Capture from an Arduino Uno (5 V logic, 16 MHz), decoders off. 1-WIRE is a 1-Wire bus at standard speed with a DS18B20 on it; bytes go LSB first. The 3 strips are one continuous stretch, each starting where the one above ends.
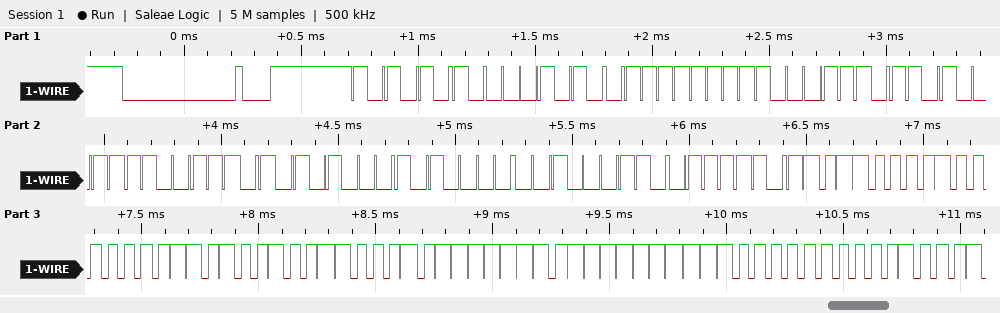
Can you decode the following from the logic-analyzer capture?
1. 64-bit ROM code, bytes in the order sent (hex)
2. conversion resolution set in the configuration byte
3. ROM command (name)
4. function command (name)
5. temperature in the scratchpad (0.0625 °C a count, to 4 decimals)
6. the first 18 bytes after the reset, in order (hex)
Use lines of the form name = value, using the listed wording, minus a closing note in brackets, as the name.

64-bit ROM code, bytes in the order sent = 28 FF 71 CB 73 15 05 62
conversion resolution set in the configuration byte = 12 bits
ROM command = Match ROM
function command = Read Scratchpad
temperature in the scratchpad = 16.8125 °C
the first 18 bytes after the reset, in order = 55 28 FF 71 CB 73 15 05 62 BE 0D 01 4B 46 7F FF 03 10
